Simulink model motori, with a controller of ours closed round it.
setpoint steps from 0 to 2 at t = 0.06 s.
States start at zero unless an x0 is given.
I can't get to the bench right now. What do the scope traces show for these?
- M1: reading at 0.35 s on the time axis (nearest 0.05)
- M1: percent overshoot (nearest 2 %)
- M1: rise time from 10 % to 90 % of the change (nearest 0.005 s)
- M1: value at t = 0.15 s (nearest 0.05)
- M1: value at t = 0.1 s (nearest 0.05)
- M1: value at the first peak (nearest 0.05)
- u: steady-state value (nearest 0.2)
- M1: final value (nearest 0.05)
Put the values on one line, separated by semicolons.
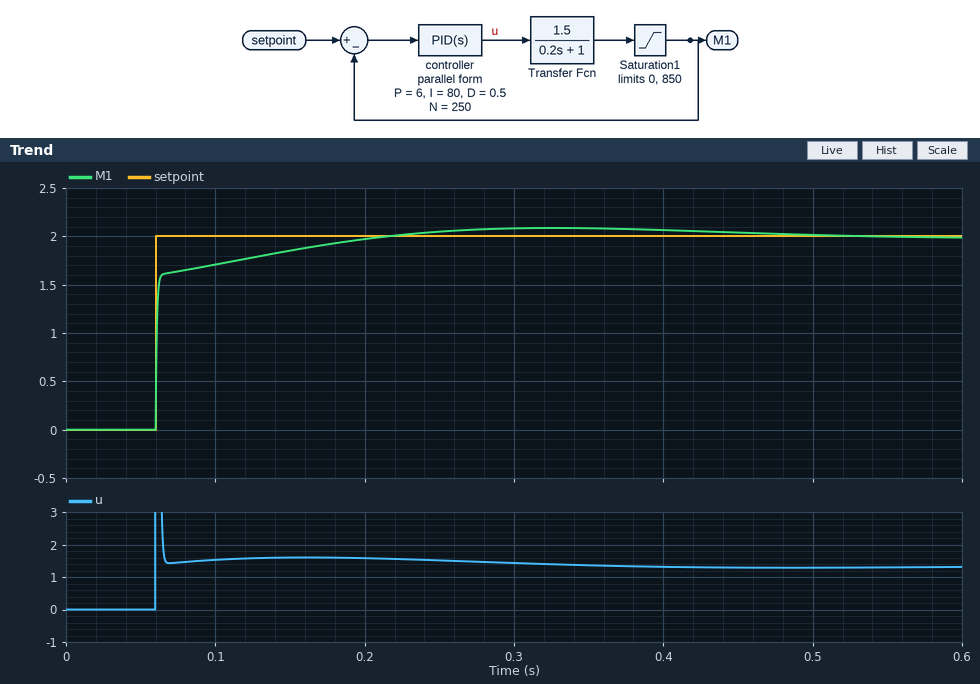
2.10; 4 %; 0.070 s; 1.85; 1.70; 2.10; 1.4; 2.00
